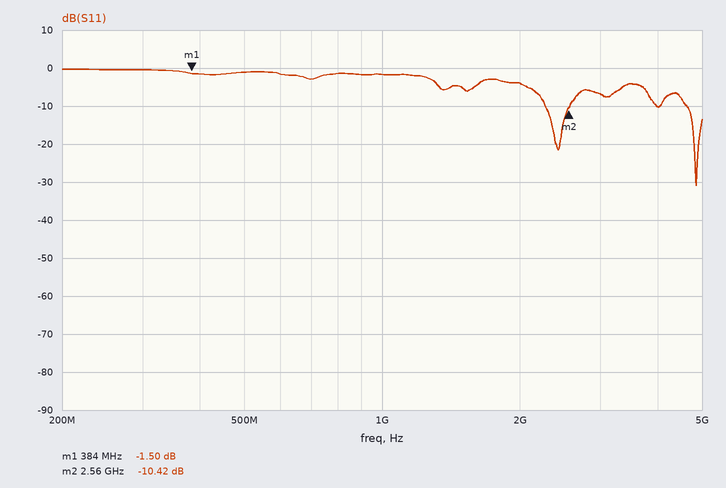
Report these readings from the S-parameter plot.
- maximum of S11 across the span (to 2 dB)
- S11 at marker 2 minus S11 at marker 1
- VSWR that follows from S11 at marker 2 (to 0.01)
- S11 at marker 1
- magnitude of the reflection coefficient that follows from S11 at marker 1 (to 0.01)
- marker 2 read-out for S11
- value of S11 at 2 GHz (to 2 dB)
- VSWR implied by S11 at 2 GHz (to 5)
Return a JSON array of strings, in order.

["0 dB", "-8.92 dB", "1.86", "-1.50 dB", "0.84", "-10.42 dB", "-4 dB", "5"]
